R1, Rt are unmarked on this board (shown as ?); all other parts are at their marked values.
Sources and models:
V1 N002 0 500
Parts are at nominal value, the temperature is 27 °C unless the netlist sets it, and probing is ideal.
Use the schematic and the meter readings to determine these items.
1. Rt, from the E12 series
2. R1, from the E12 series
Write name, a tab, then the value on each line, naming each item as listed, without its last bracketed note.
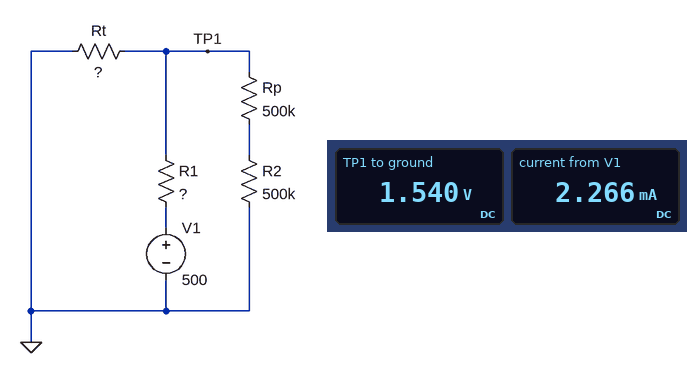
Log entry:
Rt, from the E12 series	680 Ω
R1, from the E12 series	220 kΩ
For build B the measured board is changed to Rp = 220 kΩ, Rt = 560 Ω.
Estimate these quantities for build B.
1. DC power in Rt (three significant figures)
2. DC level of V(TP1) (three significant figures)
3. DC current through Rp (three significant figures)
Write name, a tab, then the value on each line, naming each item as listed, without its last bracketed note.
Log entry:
DC power in Rt	2.87 mW
DC level of V(TP1)	1.27 V
DC current through Rp	1.76 µA
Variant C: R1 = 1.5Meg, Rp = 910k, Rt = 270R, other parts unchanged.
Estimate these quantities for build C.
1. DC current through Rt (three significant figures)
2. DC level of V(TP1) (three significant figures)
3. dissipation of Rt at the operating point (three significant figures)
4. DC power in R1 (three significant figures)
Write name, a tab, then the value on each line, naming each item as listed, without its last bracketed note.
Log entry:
DC current through Rt	333 µA
DC level of V(TP1)	90.0 mV
dissipation of Rt at the operating point	30.0 µW
DC power in R1	167 mW
